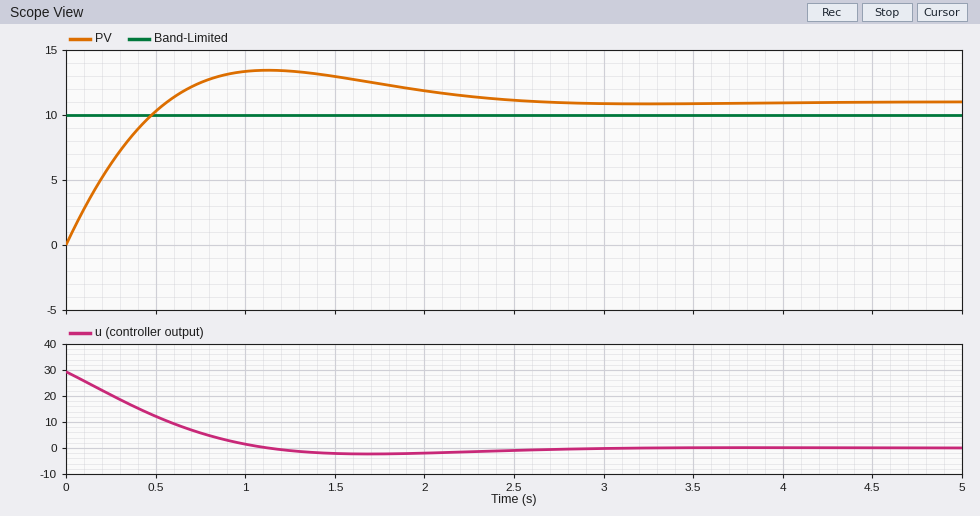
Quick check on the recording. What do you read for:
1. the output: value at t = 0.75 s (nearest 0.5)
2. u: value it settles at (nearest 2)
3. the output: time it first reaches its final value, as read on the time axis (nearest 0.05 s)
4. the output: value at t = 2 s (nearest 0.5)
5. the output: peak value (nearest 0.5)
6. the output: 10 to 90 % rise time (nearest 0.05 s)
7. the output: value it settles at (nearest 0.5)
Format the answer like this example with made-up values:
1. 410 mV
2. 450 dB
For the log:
1. 12.5
2. 0
3. 0.55 s
4. 12.0
5. 13.5
6. 0.45 s
7. 11.0
